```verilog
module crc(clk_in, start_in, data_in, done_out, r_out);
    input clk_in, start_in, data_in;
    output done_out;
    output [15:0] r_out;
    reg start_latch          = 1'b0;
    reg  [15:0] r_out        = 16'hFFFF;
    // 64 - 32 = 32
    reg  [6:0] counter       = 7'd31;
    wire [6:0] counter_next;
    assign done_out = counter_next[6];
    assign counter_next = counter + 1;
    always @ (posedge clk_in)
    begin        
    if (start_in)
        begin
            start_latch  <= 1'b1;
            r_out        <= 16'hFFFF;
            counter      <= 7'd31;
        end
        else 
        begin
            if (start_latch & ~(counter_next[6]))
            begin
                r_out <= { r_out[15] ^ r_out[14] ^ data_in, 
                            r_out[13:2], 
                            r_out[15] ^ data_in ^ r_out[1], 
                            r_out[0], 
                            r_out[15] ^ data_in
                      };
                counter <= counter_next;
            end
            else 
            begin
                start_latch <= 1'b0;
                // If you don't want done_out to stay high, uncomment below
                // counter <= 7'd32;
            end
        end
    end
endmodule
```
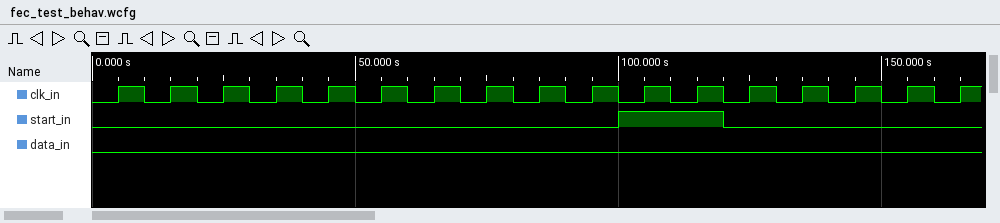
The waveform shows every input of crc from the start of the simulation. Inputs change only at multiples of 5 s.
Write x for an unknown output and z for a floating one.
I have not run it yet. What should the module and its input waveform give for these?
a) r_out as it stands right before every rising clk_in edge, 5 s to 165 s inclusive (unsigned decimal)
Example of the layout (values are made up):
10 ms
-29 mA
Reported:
65535, 65535, 65535, 65535, 65535, 65535, 65535, 65535, 65535, 65535, 65535, 65535, 65535, 32763, 65526, 32745, 65490
